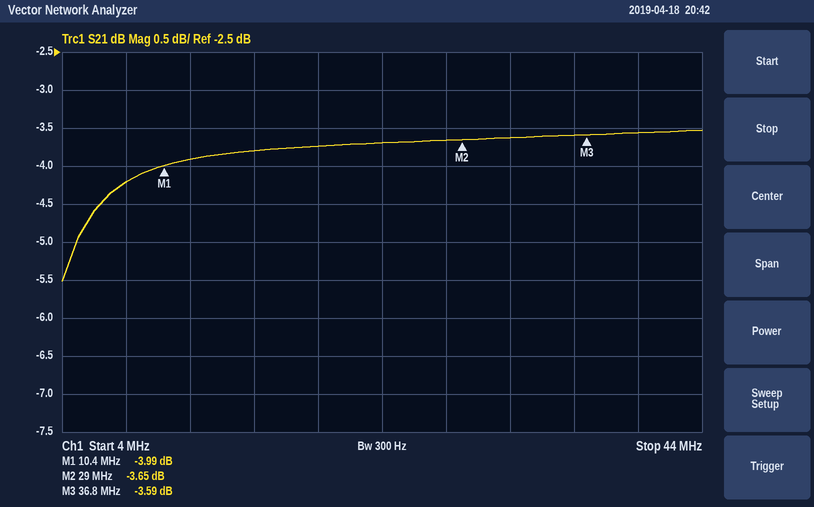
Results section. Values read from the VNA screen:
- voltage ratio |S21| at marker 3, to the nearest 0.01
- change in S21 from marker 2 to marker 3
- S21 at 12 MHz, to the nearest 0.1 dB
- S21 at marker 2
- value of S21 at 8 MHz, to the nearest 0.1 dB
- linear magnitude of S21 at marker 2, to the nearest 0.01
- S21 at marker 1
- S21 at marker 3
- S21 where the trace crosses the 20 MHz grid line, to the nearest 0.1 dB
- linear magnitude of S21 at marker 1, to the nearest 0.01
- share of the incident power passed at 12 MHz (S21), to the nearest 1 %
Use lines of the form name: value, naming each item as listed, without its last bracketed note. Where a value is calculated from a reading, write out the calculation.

voltage ratio |S21| at marker 3, to the nearest 0.01: 10^(-3.59/20) ≈ 0.66
change in S21 from marker 2 to marker 3: -3.59 − (-3.65) = 0.06 dB
S21 at 12 MHz, to the nearest 0.1 dB: -3.9 dB
S21 at marker 2: -3.65 dB
value of S21 at 8 MHz, to the nearest 0.1 dB: -4.2 dB
linear magnitude of S21 at marker 2, to the nearest 0.01: 10^(-3.65/20) ≈ 0.66
S21 at marker 1: -3.99 dB
S21 at marker 3: -3.59 dB
S21 where the trace crosses the 20 MHz grid line, to the nearest 0.1 dB: -3.7 dB
linear magnitude of S21 at marker 1, to the nearest 0.01: 10^(-3.99/20) ≈ 0.63
share of the incident power passed at 12 MHz (S21), to the nearest 1 %: 10^(-3.9/10) ≈ 41 %
